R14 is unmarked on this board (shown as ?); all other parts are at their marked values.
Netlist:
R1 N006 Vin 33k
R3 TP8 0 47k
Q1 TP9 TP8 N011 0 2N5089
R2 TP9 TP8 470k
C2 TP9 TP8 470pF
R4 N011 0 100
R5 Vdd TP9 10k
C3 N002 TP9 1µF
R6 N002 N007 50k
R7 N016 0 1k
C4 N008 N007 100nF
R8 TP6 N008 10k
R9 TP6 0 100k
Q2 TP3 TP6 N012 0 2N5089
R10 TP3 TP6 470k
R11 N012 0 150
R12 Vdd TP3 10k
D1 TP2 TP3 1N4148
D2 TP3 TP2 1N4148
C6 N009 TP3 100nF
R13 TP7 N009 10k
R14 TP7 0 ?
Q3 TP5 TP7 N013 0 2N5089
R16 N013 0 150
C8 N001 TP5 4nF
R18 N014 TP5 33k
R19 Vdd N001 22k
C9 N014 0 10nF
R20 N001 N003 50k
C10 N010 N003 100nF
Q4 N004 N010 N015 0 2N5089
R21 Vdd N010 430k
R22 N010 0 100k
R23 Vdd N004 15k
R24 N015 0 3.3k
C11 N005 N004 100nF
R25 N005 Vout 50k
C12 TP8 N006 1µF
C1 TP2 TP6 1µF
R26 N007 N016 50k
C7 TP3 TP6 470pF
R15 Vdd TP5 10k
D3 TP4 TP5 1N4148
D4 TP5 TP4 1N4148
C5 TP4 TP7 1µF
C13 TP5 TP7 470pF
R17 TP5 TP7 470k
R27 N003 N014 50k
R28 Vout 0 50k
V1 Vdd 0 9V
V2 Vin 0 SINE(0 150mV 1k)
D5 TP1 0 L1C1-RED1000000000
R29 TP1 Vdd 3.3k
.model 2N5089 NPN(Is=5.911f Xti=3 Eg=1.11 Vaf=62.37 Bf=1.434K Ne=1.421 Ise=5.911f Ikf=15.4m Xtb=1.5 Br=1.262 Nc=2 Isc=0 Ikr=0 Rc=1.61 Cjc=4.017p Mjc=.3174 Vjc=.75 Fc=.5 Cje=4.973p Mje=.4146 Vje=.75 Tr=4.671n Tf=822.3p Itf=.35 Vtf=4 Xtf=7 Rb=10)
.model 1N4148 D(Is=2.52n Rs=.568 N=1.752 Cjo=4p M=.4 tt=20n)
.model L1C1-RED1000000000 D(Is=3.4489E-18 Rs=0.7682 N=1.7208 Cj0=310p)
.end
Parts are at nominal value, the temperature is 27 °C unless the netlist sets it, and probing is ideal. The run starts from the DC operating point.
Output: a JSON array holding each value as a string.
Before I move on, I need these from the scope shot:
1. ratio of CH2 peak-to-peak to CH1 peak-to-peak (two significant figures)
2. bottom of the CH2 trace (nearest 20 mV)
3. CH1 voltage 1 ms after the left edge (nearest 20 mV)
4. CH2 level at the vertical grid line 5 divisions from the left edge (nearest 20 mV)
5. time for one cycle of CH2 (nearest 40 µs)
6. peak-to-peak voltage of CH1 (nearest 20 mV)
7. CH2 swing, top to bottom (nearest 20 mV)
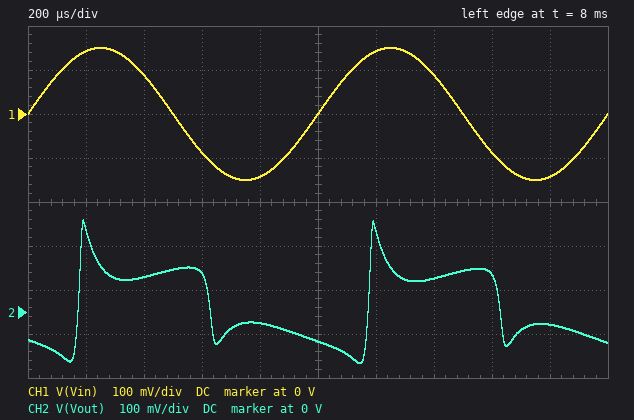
["1.1", "-120 mV", "0 V", "-60 mV", "1.00 ms", "300 mV", "320 mV"]
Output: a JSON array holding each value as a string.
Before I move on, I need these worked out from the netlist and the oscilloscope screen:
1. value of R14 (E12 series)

["33 kΩ"]
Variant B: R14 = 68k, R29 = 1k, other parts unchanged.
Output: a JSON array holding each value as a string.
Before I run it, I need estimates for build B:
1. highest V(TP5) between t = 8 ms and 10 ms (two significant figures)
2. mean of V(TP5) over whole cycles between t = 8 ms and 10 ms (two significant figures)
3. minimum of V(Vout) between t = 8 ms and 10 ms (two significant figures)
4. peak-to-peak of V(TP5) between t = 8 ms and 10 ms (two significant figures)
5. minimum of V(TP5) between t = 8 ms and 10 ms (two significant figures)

["6.1 V", "5.7 V", "-290 mV", "820 mV", "5.3 V"]
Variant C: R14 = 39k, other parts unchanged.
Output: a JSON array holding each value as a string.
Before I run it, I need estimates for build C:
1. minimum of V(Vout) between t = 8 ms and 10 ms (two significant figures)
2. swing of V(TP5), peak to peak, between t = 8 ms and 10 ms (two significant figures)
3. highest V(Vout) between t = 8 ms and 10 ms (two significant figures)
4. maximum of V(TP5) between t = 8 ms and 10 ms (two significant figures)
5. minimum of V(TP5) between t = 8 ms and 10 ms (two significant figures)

["-220 mV", "760 mV", "270 mV", "8.4 V", "7.7 V"]
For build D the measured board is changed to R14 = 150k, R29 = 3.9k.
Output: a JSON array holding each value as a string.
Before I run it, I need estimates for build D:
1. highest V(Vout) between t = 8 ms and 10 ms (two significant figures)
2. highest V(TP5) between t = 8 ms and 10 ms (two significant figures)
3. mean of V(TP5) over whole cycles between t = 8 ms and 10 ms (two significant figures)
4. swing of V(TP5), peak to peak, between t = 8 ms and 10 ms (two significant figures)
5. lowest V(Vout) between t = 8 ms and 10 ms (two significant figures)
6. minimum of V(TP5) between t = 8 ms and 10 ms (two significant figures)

["290 mV", "3.8 V", "3.4 V", "830 mV", "-300 mV", "3.0 V"]
